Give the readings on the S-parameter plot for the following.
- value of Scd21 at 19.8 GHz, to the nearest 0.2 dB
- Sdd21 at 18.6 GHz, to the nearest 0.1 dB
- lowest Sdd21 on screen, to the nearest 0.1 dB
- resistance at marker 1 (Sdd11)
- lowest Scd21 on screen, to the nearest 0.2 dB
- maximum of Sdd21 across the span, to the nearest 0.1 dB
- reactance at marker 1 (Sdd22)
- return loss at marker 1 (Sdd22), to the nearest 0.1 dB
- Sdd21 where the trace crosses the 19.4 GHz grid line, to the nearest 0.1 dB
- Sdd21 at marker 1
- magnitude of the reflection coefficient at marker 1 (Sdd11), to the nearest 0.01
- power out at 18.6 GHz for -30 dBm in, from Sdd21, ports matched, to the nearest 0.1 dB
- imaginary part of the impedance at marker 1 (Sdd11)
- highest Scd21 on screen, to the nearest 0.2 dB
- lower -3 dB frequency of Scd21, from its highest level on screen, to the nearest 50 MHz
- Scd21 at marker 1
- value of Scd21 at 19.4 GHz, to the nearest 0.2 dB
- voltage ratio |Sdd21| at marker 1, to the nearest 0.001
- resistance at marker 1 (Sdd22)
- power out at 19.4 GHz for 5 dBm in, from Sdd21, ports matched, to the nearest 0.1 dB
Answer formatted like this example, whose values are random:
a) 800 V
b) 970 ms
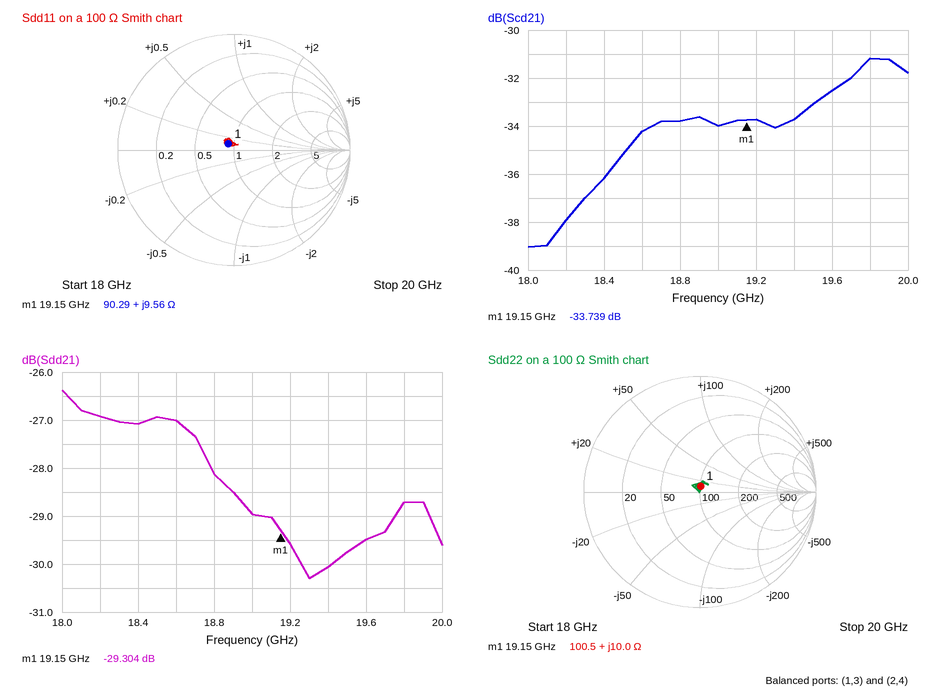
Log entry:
a) -31.2 dB
b) -27.0 dB
c) -30.3 dB
d) 90.29 Ω
e) -39.0 dB
f) -26.4 dB
g) +10.0 Ω
h) 26.0 dB
i) -30.1 dB
j) -29.304 dB
k) 0.07
l) -57.0 dBm
m) +9.56 Ω
n) -31.2 dB
o) 18.60 GHz
p) -33.739 dB
q) -33.8 dB
r) 0.034
s) 100.5 Ω
t) -25.1 dBm
